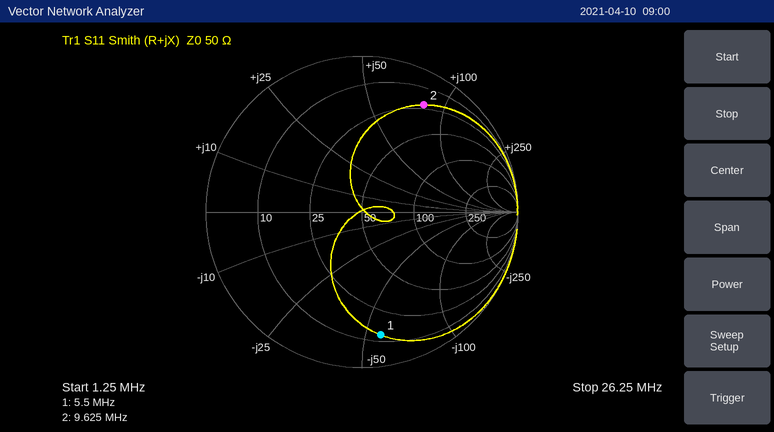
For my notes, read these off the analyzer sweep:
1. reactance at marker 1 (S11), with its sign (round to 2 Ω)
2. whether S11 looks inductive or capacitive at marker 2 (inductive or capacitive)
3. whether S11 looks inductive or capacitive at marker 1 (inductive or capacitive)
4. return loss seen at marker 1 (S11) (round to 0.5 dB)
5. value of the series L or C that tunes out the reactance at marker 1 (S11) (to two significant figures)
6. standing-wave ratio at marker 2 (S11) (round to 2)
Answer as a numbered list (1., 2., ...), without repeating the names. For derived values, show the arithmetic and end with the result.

1. -56 Ω
2. inductive
3. capacitive
4. 2.0 dB
5. L = 56 Ω/(2π × 5.5 MHz) ≈ 1.6 µH
6. 8
